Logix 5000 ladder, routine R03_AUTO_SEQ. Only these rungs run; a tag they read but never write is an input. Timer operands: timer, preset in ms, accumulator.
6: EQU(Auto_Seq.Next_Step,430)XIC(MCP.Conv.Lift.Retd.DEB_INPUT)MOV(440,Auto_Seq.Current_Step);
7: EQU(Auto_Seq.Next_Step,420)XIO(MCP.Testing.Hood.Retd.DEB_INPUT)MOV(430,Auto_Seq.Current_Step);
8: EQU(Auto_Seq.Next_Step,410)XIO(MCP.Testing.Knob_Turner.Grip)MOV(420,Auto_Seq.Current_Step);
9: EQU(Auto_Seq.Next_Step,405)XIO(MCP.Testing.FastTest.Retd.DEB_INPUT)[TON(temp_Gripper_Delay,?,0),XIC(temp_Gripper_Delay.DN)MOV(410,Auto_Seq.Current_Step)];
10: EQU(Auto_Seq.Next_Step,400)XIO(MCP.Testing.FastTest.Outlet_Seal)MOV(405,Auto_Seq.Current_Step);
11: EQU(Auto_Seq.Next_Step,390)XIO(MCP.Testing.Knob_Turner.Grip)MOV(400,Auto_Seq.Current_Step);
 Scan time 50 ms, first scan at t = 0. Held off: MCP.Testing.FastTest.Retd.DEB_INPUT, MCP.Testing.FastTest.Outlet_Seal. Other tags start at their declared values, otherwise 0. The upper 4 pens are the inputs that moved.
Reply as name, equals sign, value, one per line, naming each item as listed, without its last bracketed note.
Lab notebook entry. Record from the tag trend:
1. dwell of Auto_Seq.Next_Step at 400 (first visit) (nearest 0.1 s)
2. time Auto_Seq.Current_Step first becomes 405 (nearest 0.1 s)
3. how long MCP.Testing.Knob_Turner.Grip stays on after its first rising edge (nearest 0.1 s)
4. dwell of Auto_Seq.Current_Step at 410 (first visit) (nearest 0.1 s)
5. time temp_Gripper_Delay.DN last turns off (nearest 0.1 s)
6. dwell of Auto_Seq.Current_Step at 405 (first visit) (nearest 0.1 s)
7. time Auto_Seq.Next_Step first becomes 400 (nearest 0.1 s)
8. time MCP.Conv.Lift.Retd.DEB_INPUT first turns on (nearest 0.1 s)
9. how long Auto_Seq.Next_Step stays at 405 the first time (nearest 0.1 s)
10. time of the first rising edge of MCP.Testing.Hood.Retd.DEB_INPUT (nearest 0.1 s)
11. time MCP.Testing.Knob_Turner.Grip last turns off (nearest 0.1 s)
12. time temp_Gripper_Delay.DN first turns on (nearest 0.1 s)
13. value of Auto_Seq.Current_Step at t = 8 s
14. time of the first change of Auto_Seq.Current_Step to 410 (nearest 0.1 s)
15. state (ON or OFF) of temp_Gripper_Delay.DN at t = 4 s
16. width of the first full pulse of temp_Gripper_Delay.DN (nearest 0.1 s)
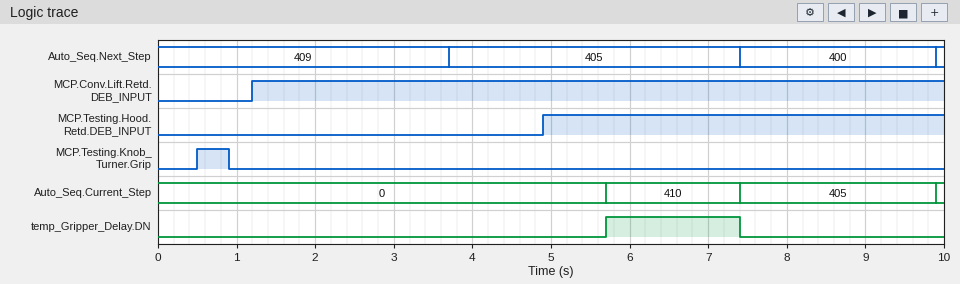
dwell of Auto_Seq.Next_Step at 400 (first visit) = 2.5 s
time Auto_Seq.Current_Step first becomes 405 = 7.4 s
how long MCP.Testing.Knob_Turner.Grip stays on after its first rising edge = 0.4 s
dwell of Auto_Seq.Current_Step at 410 (first visit) = 1.7 s
time temp_Gripper_Delay.DN last turns off = 7.4 s
dwell of Auto_Seq.Current_Step at 405 (first visit) = 2.5 s
time Auto_Seq.Next_Step first becomes 400 = 7.4 s
time MCP.Conv.Lift.Retd.DEB_INPUT first turns on = 1.2 s
how long Auto_Seq.Next_Step stays at 405 the first time = 3.7 s
time of the first rising edge of MCP.Testing.Hood.Retd.DEB_INPUT = 4.9 s
time MCP.Testing.Knob_Turner.Grip last turns off = 0.9 s
time temp_Gripper_Delay.DN first turns on = 5.7 s
value of Auto_Seq.Current_Step at t = 8 s = 405
time of the first change of Auto_Seq.Current_Step to 410 = 5.7 s
state (ON or OFF) of temp_Gripper_Delay.DN at t = 4 s = OFF
width of the first full pulse of temp_Gripper_Delay.DN = 1.7 s
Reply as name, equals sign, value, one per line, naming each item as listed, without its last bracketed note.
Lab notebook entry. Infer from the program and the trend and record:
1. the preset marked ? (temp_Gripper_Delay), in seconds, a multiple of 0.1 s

the preset marked ? (temp_Gripper_Delay), in seconds, a multiple of 0.1 s = 2.0 s
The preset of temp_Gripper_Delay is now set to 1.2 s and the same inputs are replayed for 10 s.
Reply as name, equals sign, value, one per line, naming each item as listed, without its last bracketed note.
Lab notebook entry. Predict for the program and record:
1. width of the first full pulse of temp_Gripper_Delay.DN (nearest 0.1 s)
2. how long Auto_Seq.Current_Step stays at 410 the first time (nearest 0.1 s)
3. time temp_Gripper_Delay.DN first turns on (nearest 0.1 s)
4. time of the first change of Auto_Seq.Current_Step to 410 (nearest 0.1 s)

width of the first full pulse of temp_Gripper_Delay.DN = 2.5 s
how long Auto_Seq.Current_Step stays at 410 the first time = 2.5 s
time temp_Gripper_Delay.DN first turns on = 4.9 s
time of the first change of Auto_Seq.Current_Step to 410 = 4.9 s
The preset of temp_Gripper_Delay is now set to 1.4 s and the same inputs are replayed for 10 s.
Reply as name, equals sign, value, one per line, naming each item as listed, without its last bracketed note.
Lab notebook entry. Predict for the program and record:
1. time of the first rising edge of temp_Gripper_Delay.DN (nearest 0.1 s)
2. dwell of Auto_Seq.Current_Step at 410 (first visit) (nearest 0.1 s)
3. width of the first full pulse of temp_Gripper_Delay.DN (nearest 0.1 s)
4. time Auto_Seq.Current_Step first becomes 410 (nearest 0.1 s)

time of the first rising edge of temp_Gripper_Delay.DN = 5.1 s
dwell of Auto_Seq.Current_Step at 410 (first visit) = 2.3 s
width of the first full pulse of temp_Gripper_Delay.DN = 2.3 s
time Auto_Seq.Current_Step first becomes 410 = 5.1 s
